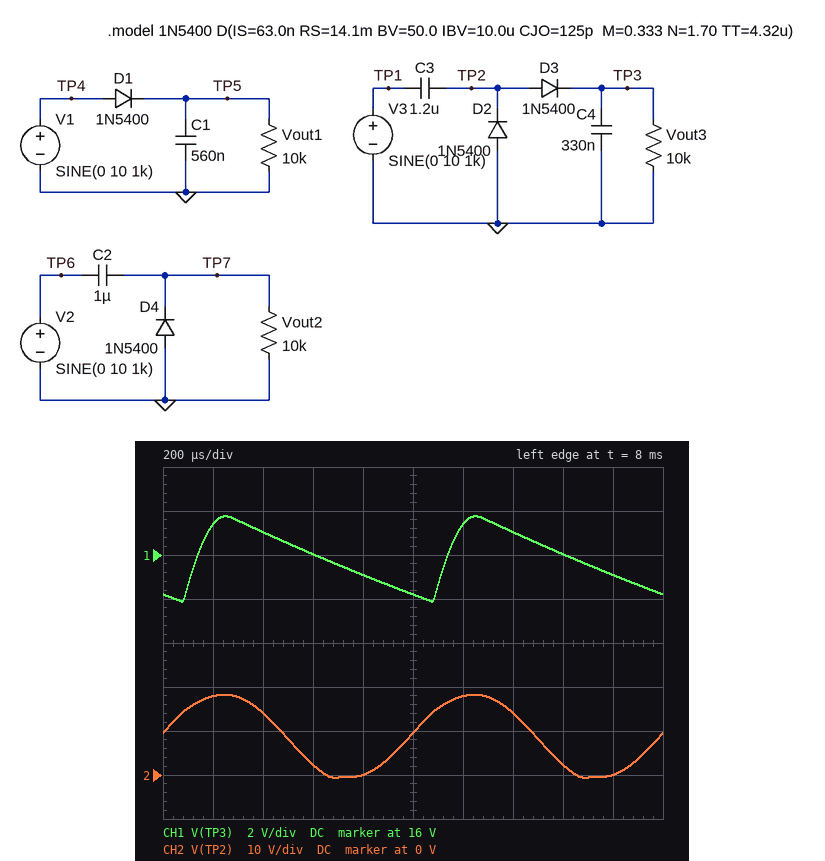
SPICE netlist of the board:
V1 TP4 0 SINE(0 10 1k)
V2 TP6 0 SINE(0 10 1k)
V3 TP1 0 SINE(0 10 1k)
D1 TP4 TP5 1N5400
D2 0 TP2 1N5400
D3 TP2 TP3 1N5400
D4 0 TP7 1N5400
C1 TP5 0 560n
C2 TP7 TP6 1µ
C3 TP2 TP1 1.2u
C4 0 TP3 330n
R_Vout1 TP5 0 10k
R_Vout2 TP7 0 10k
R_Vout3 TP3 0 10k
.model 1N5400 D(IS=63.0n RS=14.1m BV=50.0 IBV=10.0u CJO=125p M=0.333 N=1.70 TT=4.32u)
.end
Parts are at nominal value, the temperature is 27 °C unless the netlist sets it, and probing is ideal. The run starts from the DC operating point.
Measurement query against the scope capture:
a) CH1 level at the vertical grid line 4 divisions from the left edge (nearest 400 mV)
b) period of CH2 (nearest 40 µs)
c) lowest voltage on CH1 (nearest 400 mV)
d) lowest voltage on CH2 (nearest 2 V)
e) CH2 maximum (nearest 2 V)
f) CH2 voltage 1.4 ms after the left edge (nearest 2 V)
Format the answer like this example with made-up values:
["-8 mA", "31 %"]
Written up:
["15.2 V", "1.00 ms", "14.0 V", "0 V", "18 V", "14 V"]
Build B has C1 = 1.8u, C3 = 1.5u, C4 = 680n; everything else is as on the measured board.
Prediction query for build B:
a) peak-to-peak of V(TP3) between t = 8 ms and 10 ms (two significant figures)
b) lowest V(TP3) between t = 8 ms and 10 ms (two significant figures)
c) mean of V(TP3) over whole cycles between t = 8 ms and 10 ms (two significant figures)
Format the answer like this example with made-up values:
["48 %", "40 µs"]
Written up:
["2.1 V", "16 V", "17 V"]
